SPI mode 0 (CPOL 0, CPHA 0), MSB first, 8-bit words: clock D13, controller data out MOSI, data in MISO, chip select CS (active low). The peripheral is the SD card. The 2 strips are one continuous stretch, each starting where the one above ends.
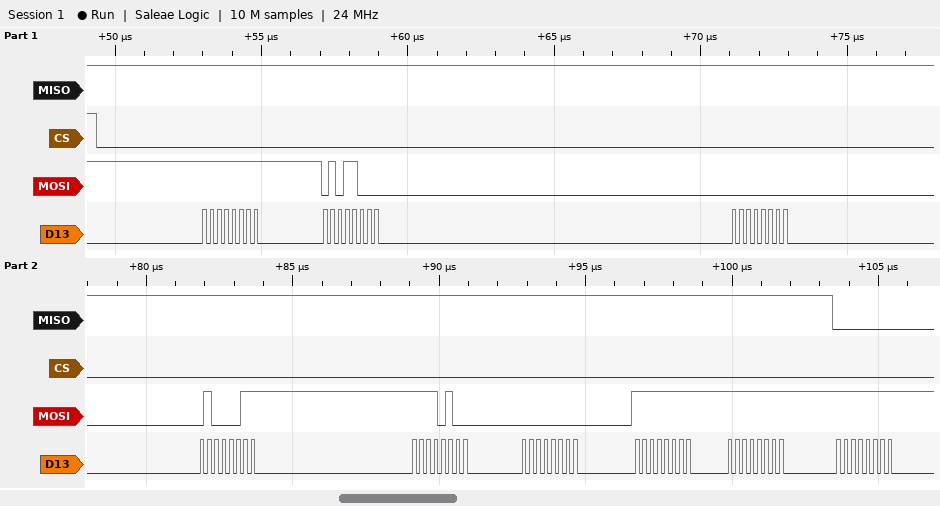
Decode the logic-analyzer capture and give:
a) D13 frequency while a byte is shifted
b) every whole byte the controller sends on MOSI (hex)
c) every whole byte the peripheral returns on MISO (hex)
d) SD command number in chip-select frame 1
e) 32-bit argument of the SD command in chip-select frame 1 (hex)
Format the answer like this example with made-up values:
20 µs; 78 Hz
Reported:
4 MHz; 0xFF 0x58 0x00 0x43 0xF4 0x00 0xFF 0xFF 0xFF; 0xFF 0xFF 0xFF 0xFF 0xFF 0xFF 0xFF 0xFF 0x00; CMD24; 0x0043F400
